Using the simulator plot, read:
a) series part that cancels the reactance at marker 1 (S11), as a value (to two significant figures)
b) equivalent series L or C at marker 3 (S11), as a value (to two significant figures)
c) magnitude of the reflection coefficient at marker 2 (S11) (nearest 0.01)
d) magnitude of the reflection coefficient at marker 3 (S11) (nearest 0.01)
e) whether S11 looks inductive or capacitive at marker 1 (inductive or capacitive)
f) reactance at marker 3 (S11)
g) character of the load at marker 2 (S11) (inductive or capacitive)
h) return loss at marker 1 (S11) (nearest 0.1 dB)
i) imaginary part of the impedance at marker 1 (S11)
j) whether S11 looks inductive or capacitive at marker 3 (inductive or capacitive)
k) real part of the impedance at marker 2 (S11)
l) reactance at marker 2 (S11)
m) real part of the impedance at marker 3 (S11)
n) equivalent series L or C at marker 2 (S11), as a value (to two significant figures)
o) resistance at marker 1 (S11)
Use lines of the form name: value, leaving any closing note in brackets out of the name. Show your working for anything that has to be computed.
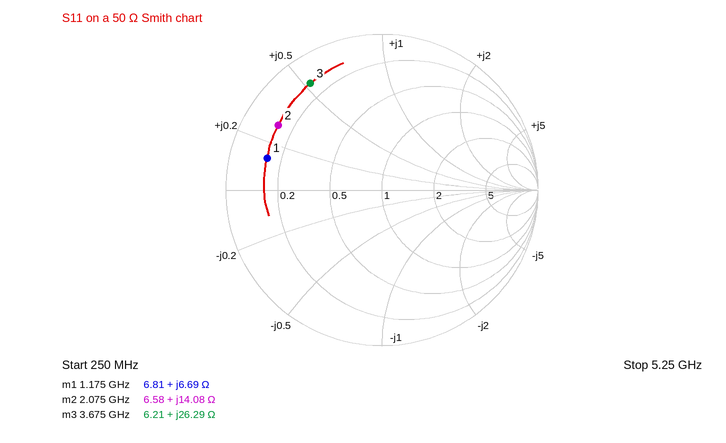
series part that cancels the reactance at marker 1 (S11), as a value: C = 1/(2π × 1.175 GHz × 6.69 Ω) ≈ 20 pF
equivalent series L or C at marker 3 (S11), as a value: L = 26.29 Ω/(2π × 3.675 GHz) ≈ 1.1 nH
magnitude of the reflection coefficient at marker 2 (S11): 0.78
magnitude of the reflection coefficient at marker 3 (S11): 0.82
whether S11 looks inductive or capacitive at marker 1: inductive
reactance at marker 3: +26.29 Ω
character of the load at marker 2 (S11): inductive
return loss at marker 1 (S11): 2.3 dB
imaginary part of the impedance at marker 1: +6.69 Ω
whether S11 looks inductive or capacitive at marker 3: inductive
real part of the impedance at marker 2: 6.58 Ω
reactance at marker 2: +14.08 Ω
real part of the impedance at marker 3: 6.21 Ω
equivalent series L or C at marker 2 (S11), as a value: L = 14.08 Ω/(2π × 2.075 GHz) ≈ 1.1 nH
resistance at marker 1: 6.81 Ω
